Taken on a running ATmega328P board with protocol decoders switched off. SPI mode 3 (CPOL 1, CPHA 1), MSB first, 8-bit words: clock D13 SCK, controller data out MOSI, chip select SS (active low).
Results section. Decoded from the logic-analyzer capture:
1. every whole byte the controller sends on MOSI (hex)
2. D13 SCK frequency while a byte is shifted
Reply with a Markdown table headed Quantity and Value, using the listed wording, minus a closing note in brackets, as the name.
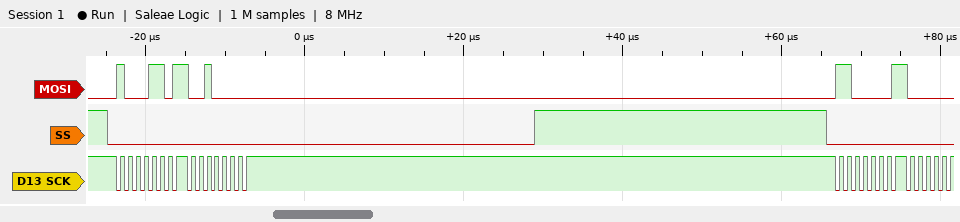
| Quantity | Value |
|---|---|
| every whole byte the controller sends on MOSI | 0x8D 0x20 0xC1 |
| D13 SCK frequency while a byte is shifted | 1 MHz |
